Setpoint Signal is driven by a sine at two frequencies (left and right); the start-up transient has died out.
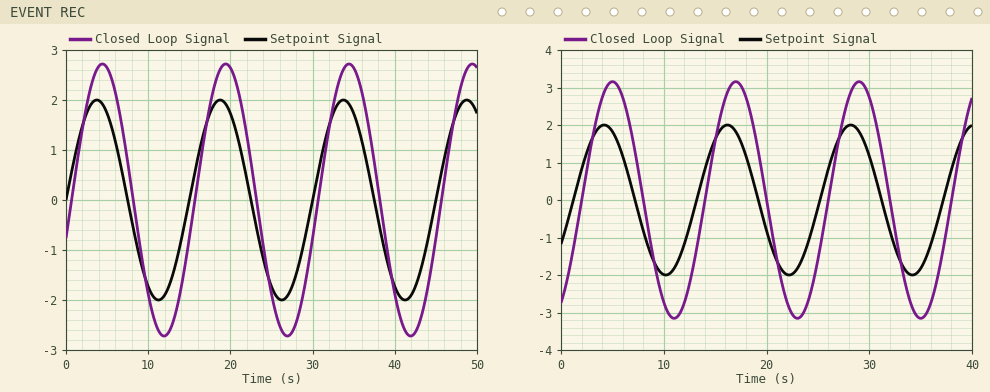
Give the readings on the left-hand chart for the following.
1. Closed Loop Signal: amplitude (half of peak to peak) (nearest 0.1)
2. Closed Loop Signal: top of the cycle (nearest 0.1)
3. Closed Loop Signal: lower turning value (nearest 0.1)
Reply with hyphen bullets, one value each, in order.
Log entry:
- 2.7
- 2.7
- -2.7
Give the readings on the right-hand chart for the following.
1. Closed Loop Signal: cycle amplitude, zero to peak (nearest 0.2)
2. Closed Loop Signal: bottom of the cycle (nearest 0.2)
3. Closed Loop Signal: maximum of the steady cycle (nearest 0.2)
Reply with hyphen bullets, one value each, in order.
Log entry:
- 3.2
- -3.2
- 3.2
